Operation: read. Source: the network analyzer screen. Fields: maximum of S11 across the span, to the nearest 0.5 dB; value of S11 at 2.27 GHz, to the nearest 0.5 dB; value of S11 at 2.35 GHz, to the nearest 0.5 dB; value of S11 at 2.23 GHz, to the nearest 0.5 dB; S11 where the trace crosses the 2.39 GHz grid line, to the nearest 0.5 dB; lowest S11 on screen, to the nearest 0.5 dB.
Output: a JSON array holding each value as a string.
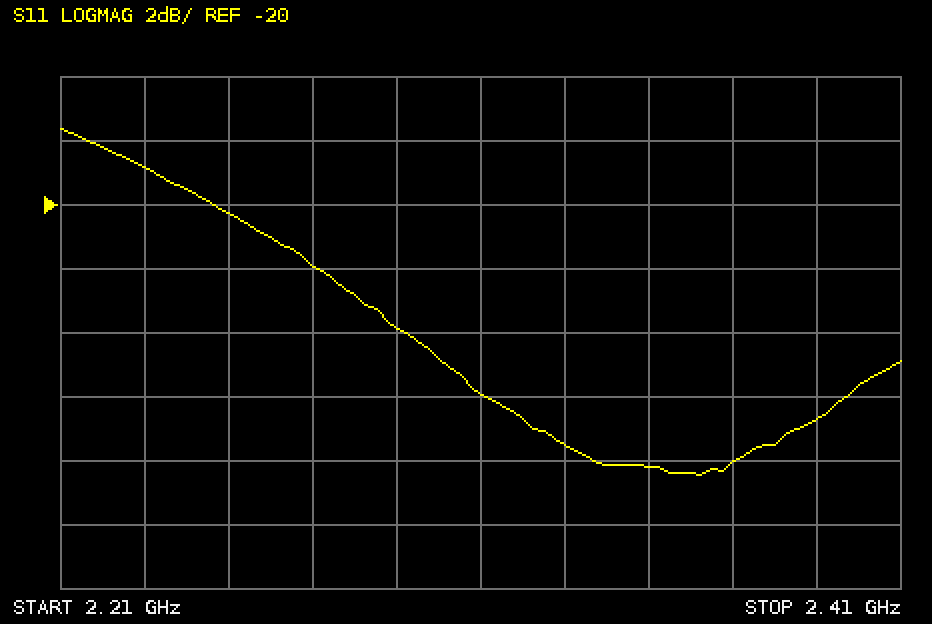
["-17.5 dB", "-22.0 dB", "-28.0 dB", "-19.0 dB", "-26.5 dB", "-28.5 dB"]
